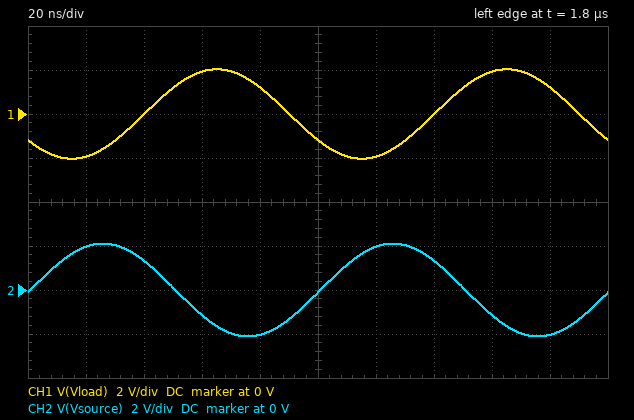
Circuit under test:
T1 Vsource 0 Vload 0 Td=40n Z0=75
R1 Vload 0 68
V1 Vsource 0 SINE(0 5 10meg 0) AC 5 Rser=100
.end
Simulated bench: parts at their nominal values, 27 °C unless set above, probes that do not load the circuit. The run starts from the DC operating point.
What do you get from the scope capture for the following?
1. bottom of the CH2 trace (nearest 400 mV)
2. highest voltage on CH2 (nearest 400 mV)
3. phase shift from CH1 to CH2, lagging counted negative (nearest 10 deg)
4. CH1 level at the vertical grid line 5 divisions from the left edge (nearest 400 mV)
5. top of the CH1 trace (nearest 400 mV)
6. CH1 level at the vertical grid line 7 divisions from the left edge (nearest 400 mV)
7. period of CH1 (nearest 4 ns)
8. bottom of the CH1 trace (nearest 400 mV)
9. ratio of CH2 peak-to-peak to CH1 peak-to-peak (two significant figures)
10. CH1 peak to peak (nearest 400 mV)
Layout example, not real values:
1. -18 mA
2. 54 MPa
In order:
1. -2.0 V
2. 2.0 V
3. 140 deg
4. -1.2 V
5. 2.0 V
6. 0 V
7. 100 ns
8. -2.0 V
9. 1.0
10. 4.0 V
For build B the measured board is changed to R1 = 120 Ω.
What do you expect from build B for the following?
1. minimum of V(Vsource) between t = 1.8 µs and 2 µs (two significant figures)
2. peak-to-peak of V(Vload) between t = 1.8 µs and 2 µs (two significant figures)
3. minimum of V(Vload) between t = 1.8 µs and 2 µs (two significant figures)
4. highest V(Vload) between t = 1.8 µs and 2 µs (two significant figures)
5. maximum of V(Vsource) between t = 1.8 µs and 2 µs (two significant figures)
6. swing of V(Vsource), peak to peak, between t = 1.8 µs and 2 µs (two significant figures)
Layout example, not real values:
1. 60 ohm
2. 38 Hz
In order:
1. -2.4 V
2. 5.3 V
3. -2.7 V
4. 2.7 V
5. 2.4 V
6. 4.7 V
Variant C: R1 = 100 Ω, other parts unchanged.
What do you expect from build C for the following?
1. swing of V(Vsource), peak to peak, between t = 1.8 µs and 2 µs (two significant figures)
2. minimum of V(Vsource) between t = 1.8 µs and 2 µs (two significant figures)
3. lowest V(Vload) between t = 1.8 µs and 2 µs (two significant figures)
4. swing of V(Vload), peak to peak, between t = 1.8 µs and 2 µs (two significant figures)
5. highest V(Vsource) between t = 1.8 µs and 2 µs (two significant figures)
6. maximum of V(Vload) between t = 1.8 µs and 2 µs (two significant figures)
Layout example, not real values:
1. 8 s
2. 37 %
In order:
1. 4.5 V
2. -2.3 V
3. -2.5 V
4. 4.9 V
5. 2.3 V
6. 2.5 V
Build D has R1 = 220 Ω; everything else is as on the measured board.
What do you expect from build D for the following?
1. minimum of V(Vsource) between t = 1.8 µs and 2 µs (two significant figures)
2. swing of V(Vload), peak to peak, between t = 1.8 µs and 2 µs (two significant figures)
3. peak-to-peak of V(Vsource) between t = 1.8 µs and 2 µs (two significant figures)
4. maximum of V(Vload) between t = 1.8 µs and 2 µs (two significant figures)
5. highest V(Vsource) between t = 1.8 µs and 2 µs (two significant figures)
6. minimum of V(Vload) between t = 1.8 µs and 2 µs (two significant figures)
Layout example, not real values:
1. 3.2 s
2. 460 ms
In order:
1. -2.7 V
2. 6.5 V
3. 5.4 V
4. 3.3 V
5. 2.7 V
6. -3.3 V
